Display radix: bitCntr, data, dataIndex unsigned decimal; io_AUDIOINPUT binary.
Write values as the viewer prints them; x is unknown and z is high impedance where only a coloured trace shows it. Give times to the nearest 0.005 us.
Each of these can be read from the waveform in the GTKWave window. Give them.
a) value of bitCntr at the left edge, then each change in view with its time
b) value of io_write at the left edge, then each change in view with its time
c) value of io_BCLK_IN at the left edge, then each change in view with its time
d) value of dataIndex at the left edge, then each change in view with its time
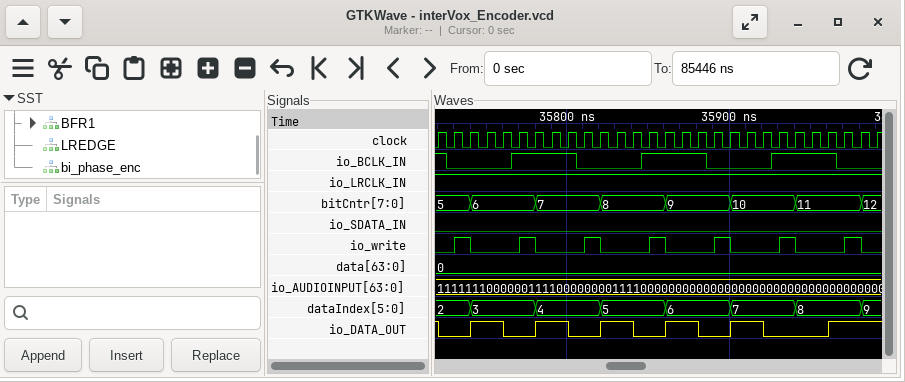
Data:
5, 6 at 35.74 us, 7 at 35.78 us, 8 at 35.82 us, 9 at 35.86 us, 10 at 35.9 us, 11 at 35.94 us, 12 at 35.98 us
0, 1 at 35.73 us, 0 at 35.74 us, 1 at 35.77 us, 0 at 35.78 us, 1 at 35.81 us, 0 at 35.82 us, 1 at 35.85 us, 0 at 35.86 us, 1 at 35.89 us, 0 at 35.9 us, 1 at 35.93 us, 0 at 35.94 us, 1 at 35.97 us, 0 at 35.98 us
1, 0 at 35.725 us, 1 at 35.765 us, 0 at 35.805 us, 1 at 35.845 us, 0 at 35.885 us, 1 at 35.925 us, 0 at 35.965 us
2, 3 at 35.74 us, 4 at 35.78 us, 5 at 35.82 us, 6 at 35.86 us, 7 at 35.9 us, 8 at 35.94 us, 9 at 35.98 us
